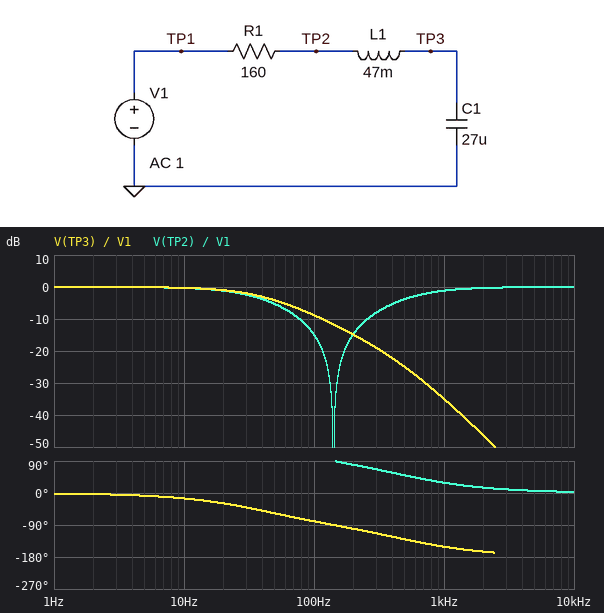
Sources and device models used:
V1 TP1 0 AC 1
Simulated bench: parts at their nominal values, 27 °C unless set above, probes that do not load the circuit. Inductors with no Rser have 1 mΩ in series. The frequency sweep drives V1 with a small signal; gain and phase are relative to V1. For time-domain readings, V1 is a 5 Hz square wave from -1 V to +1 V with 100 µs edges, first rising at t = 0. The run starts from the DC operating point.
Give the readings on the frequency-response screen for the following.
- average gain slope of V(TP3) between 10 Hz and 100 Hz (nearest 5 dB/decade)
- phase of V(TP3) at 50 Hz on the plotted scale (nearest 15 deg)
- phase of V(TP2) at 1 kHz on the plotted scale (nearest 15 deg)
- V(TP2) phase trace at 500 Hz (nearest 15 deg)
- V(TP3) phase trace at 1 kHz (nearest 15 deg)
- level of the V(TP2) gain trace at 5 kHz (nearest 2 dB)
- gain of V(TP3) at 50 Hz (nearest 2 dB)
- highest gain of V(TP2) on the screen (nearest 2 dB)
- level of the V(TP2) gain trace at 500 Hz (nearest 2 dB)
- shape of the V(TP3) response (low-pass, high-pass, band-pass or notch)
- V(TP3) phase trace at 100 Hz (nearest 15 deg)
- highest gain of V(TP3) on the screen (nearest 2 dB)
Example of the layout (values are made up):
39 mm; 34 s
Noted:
-10 dB/decade; -60 deg; 30 deg; 45 deg; -150 deg; 0 dB; -4 dB; 0 dB; -4 dB; low-pass; -75 deg; 0 dB
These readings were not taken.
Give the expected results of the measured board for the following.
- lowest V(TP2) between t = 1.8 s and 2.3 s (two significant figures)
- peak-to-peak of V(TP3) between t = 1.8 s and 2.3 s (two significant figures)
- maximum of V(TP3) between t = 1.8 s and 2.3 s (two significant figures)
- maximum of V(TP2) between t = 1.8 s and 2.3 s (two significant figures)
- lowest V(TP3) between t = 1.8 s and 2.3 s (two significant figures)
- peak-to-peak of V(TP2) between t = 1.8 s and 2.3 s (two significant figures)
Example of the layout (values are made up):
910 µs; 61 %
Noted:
-1.0 V; 2.0 V; 1.0 V; 1.0 V; -1.0 V; 2.0 V
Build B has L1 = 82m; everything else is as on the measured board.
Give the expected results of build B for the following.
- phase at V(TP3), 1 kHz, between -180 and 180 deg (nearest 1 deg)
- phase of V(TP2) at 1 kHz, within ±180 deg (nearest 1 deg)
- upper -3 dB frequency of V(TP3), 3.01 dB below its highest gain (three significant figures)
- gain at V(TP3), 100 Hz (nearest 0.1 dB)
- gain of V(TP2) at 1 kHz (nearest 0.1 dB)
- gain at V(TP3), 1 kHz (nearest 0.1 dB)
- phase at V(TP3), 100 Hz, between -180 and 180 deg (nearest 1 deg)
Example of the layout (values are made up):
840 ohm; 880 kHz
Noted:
-163 deg; 17 deg; 41.7 Hz; -8.7 dB; -0.4 dB; -39.1 dB; -87 deg
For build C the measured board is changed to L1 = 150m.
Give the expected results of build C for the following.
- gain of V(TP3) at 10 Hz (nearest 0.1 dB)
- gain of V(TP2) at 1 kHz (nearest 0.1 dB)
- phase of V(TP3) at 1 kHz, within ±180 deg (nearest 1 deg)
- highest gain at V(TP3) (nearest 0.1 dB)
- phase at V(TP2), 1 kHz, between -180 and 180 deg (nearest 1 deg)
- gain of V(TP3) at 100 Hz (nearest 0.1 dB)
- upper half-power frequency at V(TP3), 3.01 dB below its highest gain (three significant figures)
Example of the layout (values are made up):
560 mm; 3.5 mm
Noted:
-0.2 dB; -0.1 dB; -170 deg; 0 dB; 10 deg; -8.9 dB; 46.1 Hz
